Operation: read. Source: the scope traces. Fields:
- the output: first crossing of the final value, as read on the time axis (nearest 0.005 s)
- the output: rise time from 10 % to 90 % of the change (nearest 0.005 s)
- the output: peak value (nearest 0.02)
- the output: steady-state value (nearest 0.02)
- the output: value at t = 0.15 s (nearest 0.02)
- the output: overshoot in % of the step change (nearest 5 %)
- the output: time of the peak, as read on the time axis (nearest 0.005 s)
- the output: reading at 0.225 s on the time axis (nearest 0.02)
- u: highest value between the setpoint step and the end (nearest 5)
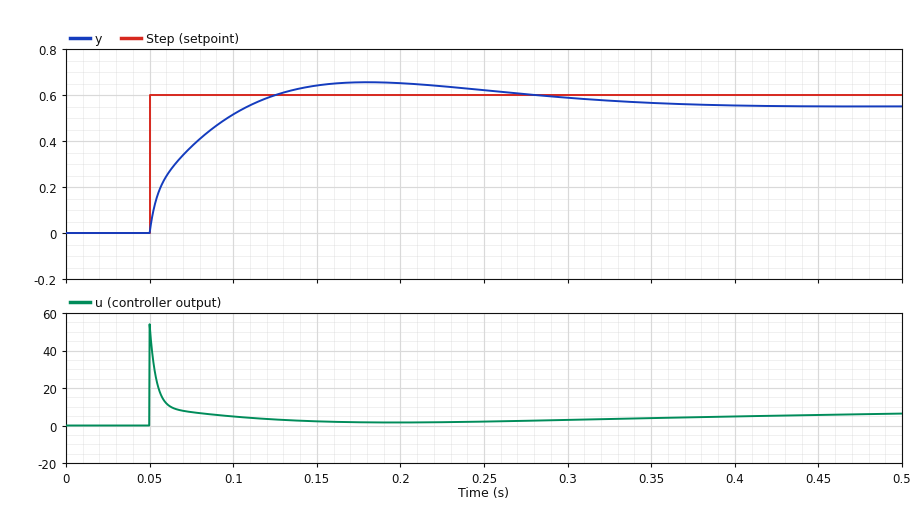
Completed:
0.110 s
0.045 s
0.66
0.56
0.64
20 %
0.180 s
0.64
55
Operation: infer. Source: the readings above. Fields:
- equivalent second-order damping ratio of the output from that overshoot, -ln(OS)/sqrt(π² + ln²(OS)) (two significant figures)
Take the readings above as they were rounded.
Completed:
0.46
